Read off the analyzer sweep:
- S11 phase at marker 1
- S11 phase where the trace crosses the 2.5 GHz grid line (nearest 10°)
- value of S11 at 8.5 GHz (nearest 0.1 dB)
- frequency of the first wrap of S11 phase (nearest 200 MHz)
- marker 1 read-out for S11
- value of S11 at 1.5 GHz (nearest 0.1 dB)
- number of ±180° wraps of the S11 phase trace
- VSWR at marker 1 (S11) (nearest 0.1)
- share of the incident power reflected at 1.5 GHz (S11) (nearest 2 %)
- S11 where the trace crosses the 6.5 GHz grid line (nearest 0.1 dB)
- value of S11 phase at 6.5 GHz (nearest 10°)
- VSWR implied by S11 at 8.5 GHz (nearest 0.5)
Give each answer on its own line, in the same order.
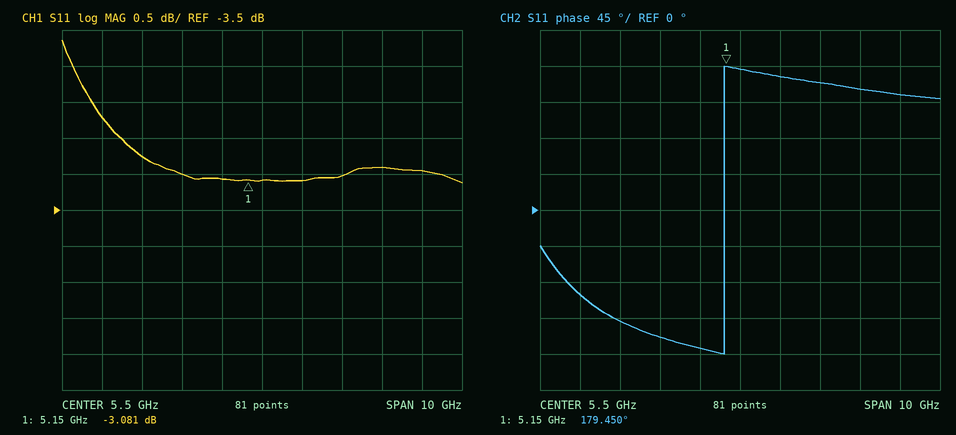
179.450°
-140°
-2.9 dB
5.2 GHz
-3.081 dB
-2.2 dB
1
5.7
60 %
-3.1 dB
170°
6.0
